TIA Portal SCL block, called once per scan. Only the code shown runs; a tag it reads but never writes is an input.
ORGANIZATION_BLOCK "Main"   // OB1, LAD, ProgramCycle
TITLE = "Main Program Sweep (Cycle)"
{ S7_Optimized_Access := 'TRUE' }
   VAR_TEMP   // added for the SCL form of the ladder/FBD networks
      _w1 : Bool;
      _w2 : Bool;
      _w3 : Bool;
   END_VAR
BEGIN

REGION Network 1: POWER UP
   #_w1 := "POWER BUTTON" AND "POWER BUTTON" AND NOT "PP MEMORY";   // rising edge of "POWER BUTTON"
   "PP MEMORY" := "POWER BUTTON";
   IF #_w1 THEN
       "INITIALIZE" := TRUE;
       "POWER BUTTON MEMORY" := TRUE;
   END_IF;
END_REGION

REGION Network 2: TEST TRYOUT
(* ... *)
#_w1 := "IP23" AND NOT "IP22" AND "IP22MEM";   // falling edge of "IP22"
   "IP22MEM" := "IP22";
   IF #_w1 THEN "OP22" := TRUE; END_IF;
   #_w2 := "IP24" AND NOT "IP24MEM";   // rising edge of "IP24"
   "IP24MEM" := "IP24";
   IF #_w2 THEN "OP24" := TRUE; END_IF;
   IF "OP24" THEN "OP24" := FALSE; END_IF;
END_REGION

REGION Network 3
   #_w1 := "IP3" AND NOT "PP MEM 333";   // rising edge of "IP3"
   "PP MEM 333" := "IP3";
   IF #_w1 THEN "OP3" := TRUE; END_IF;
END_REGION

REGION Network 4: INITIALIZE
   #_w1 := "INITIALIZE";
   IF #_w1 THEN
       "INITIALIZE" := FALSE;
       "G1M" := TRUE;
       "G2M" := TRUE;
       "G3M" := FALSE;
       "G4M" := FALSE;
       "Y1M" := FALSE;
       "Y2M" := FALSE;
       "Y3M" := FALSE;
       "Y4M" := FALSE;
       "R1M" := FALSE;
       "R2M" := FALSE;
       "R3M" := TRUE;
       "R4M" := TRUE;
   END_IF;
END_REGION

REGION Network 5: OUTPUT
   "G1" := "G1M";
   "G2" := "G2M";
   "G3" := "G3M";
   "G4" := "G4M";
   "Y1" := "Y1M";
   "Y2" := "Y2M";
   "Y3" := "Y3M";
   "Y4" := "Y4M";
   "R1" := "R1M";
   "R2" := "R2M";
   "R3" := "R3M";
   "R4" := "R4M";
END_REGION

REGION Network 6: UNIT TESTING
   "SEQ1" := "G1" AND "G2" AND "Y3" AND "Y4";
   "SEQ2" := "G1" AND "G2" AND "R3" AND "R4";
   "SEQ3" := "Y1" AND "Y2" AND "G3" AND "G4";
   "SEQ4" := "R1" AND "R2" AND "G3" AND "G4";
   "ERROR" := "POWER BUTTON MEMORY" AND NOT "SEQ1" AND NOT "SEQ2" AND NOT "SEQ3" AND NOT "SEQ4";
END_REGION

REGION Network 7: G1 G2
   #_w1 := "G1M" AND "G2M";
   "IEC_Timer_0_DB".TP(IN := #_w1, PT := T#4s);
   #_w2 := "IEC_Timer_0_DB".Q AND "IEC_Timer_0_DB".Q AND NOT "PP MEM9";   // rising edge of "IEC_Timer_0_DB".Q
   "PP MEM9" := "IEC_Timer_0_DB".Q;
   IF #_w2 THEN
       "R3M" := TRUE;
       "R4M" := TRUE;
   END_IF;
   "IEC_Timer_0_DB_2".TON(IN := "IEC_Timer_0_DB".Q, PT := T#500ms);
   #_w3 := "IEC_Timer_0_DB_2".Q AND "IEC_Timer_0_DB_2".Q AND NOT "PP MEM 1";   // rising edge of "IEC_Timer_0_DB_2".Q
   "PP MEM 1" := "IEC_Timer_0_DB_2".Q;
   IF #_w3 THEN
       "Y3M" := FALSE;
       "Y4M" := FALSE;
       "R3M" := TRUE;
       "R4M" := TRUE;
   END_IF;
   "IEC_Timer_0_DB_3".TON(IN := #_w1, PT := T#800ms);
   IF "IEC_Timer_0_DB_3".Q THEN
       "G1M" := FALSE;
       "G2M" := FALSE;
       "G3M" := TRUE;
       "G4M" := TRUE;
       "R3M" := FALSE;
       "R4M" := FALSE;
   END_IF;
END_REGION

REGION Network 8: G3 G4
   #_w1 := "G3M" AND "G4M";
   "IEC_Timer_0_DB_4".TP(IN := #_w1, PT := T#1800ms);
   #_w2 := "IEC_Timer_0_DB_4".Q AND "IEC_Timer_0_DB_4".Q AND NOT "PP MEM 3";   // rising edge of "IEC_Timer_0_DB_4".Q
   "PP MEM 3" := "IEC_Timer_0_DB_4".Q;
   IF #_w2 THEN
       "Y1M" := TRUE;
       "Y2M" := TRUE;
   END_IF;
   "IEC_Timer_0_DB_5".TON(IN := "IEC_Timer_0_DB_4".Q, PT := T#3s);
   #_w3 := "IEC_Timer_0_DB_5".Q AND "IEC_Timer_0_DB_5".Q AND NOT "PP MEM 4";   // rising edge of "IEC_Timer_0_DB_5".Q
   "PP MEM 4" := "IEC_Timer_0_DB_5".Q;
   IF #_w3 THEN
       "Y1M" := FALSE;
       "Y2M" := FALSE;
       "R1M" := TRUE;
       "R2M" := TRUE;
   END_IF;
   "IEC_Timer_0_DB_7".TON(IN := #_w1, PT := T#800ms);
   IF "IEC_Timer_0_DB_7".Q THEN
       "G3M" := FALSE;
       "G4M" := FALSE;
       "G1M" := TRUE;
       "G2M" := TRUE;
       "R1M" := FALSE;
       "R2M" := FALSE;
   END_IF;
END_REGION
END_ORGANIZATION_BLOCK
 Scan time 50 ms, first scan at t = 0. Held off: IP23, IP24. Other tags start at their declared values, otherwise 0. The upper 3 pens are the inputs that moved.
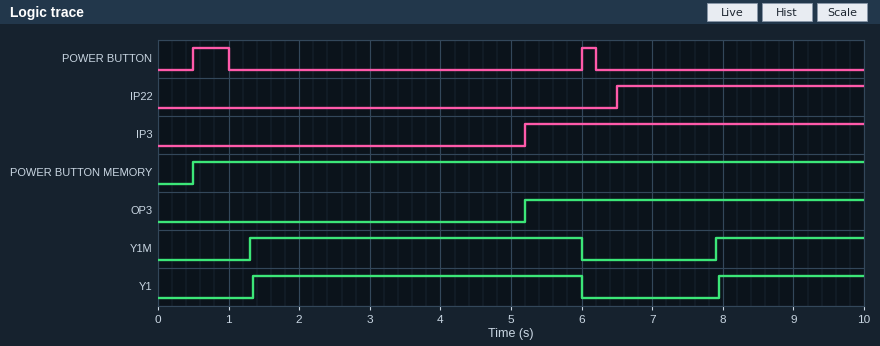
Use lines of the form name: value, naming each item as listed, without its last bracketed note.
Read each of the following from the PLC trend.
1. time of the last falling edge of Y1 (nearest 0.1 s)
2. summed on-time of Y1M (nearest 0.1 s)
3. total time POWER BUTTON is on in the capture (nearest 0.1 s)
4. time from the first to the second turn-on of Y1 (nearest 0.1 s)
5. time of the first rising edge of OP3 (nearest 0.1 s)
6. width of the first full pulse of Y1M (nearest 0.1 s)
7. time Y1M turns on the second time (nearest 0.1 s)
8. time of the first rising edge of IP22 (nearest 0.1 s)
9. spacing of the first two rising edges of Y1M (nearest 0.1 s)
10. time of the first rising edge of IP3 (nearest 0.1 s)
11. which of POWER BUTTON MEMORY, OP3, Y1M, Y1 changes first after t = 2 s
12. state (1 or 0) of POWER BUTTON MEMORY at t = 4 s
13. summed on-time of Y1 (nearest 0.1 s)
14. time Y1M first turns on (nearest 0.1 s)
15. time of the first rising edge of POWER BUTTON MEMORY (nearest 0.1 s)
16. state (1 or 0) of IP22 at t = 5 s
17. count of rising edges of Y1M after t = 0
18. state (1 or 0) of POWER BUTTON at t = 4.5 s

time of the last falling edge of Y1: 6.0 s
summed on-time of Y1M: 6.8 s
total time POWER BUTTON is on in the capture: 0.7 s
time from the first to the second turn-on of Y1: 6.6 s
time of the first rising edge of OP3: 5.2 s
width of the first full pulse of Y1M: 4.7 s
time Y1M turns on the second time: 7.9 s
time of the first rising edge of IP22: 6.5 s
spacing of the first two rising edges of Y1M: 6.6 s
time of the first rising edge of IP3: 5.2 s
which of POWER BUTTON MEMORY, OP3, Y1M, Y1 changes first after t = 2 s: OP3
state (1 or 0) of POWER BUTTON MEMORY at t = 4 s: 1
summed on-time of Y1: 6.7 s
time Y1M first turns on: 1.3 s
time of the first rising edge of POWER BUTTON MEMORY: 0.5 s
state (1 or 0) of IP22 at t = 5 s: 0
count of rising edges of Y1M after t = 0: 2
state (1 or 0) of POWER BUTTON at t = 4.5 s: 0
